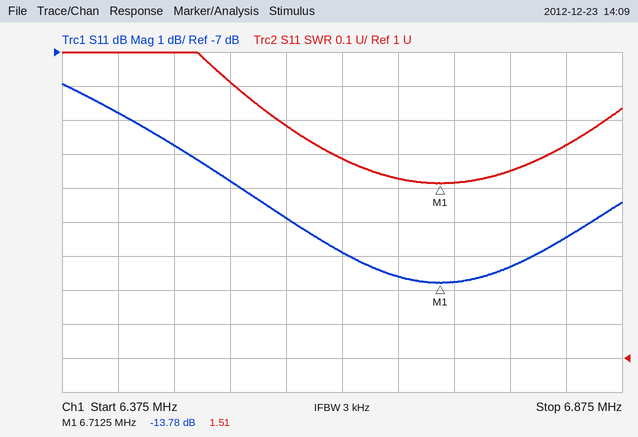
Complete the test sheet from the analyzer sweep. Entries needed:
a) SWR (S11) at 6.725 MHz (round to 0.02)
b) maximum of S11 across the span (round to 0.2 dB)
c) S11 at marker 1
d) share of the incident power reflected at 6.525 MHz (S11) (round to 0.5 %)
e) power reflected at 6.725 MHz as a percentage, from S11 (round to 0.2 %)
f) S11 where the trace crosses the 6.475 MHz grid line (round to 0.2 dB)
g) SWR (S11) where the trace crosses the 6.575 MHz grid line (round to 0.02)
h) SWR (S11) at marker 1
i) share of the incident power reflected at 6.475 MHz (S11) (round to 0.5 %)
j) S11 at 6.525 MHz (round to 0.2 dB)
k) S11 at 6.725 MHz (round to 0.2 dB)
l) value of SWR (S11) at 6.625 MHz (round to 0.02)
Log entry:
1.52
-8.0 dB
-13.78 dB
8.5 %
4.2 %
-9.8 dB
1.68
1.51
10.5 %
-10.8 dB
-13.8 dB
1.58
